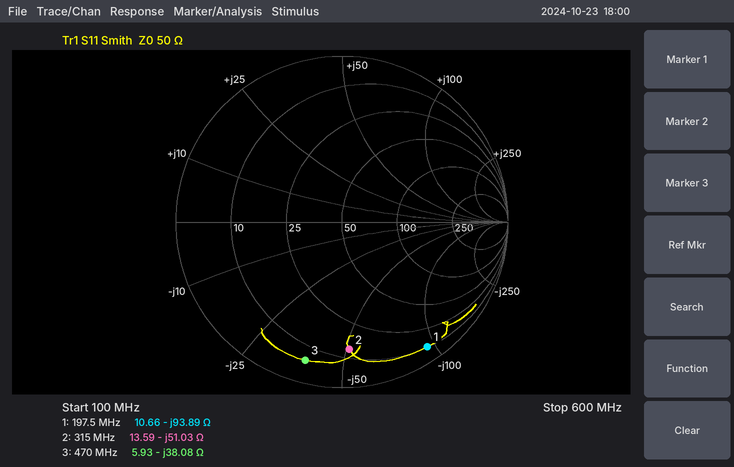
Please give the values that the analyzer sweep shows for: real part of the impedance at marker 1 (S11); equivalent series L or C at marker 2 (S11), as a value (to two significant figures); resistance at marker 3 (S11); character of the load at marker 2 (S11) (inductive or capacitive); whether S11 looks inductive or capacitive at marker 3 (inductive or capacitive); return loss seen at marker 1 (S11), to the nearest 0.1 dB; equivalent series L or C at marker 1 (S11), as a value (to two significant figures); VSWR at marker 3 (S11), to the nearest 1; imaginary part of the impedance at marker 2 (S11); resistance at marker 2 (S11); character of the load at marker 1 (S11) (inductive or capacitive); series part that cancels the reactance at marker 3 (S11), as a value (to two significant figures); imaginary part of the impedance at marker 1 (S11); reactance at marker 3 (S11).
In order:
10.66 Ω
9.9 pF
5.93 Ω
capacitive
capacitive
0.8 dB
8.6 pF
13
-51.03 Ω
13.59 Ω
capacitive
13 nH
-93.89 Ω
-38.08 Ω
